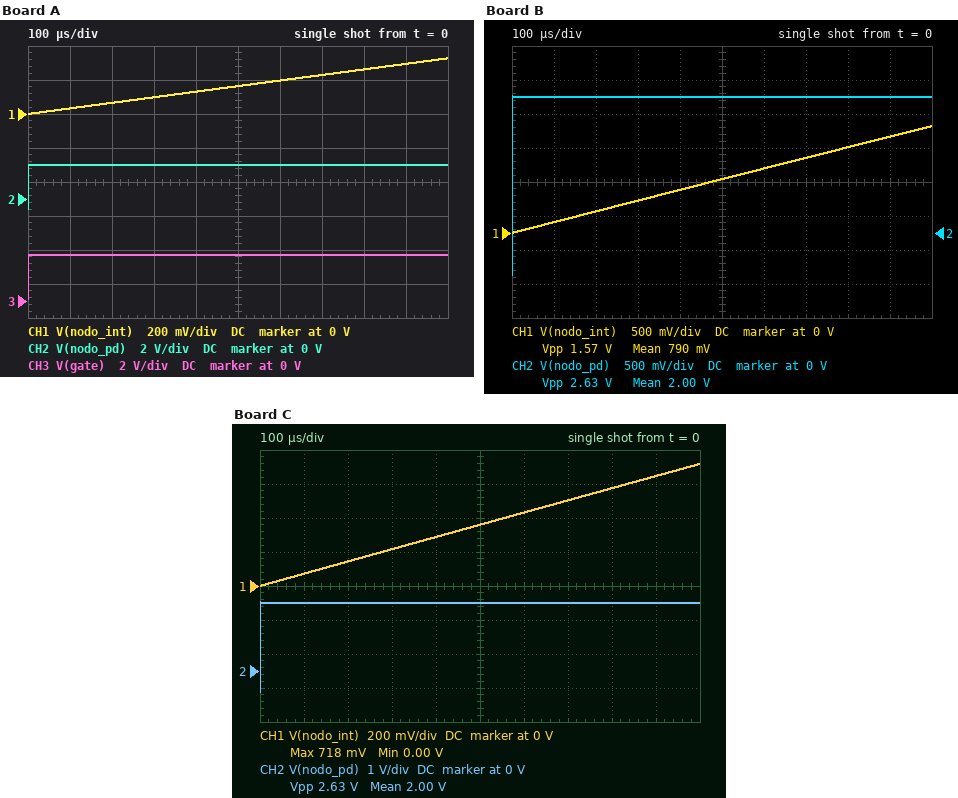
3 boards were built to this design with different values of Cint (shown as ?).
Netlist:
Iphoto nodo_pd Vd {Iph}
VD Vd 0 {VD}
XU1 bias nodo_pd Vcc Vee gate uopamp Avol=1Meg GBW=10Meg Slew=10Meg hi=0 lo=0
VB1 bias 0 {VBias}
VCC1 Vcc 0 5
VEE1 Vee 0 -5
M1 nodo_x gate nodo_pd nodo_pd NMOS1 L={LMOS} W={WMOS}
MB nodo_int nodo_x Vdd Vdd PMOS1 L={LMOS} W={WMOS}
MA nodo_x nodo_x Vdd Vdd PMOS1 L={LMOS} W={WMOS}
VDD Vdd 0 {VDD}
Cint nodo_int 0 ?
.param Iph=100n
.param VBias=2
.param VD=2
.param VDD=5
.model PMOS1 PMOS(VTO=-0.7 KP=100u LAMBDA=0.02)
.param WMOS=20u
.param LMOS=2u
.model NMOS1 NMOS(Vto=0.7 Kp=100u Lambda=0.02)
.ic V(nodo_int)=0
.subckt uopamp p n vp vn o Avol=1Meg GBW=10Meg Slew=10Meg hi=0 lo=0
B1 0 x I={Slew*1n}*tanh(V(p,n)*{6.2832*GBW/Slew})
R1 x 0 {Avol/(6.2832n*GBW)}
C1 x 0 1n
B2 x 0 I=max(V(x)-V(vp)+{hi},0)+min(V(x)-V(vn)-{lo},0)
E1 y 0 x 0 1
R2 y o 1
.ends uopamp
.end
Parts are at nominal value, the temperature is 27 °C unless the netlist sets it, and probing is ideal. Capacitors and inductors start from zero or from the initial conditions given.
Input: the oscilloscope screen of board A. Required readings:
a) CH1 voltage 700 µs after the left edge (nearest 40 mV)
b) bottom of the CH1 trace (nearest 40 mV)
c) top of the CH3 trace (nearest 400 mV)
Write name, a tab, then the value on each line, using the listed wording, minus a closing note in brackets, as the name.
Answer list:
CH1 voltage 700 µs after the left edge	240 mV
bottom of the CH1 trace	0 V
top of the CH3 trace	2.8 V
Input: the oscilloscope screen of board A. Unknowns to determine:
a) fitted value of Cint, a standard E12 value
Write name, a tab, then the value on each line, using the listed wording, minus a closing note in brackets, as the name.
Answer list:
fitted value of Cint, a standard E12 value	330 pF
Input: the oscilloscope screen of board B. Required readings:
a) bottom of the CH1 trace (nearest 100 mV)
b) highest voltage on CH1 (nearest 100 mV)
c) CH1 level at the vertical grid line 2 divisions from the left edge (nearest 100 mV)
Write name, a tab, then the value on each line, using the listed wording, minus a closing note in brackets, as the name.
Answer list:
bottom of the CH1 trace	0 V
highest voltage on CH1	1.6 V
CH1 level at the vertical grid line 2 divisions from the left edge	300 mV
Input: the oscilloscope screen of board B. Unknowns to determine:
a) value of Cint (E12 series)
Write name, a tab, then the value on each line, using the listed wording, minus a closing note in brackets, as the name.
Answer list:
value of Cint	68 pF
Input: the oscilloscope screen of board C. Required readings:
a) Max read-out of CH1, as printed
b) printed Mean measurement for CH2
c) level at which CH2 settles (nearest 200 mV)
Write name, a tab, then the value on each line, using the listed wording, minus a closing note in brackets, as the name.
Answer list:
Max read-out of CH1, as printed	718 mV
printed Mean measurement for CH2	2.00 V
level at which CH2 settles	2.0 V
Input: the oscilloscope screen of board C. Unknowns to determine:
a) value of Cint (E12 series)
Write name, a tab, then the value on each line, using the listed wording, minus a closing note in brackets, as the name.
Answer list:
value of Cint	150 pF
